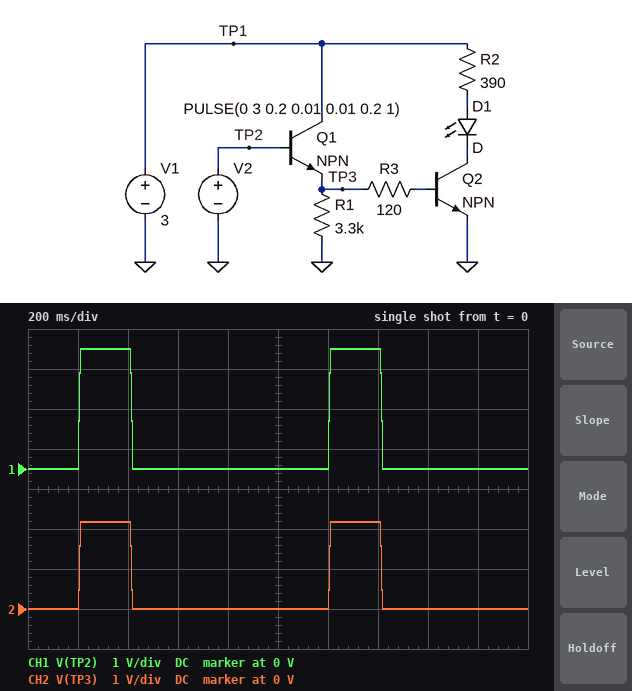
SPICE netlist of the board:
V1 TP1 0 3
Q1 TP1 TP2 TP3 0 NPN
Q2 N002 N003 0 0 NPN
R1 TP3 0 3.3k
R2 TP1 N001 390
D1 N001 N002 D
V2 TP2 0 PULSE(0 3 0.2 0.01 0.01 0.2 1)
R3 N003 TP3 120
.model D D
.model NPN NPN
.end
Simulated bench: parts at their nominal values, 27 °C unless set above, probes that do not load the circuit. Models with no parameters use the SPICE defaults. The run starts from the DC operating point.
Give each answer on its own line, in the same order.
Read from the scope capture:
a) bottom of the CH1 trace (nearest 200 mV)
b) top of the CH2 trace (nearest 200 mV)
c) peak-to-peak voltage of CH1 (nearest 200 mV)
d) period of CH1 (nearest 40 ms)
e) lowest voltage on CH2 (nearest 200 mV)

0 V
2.2 V
3.0 V
1.00 s
0 V
